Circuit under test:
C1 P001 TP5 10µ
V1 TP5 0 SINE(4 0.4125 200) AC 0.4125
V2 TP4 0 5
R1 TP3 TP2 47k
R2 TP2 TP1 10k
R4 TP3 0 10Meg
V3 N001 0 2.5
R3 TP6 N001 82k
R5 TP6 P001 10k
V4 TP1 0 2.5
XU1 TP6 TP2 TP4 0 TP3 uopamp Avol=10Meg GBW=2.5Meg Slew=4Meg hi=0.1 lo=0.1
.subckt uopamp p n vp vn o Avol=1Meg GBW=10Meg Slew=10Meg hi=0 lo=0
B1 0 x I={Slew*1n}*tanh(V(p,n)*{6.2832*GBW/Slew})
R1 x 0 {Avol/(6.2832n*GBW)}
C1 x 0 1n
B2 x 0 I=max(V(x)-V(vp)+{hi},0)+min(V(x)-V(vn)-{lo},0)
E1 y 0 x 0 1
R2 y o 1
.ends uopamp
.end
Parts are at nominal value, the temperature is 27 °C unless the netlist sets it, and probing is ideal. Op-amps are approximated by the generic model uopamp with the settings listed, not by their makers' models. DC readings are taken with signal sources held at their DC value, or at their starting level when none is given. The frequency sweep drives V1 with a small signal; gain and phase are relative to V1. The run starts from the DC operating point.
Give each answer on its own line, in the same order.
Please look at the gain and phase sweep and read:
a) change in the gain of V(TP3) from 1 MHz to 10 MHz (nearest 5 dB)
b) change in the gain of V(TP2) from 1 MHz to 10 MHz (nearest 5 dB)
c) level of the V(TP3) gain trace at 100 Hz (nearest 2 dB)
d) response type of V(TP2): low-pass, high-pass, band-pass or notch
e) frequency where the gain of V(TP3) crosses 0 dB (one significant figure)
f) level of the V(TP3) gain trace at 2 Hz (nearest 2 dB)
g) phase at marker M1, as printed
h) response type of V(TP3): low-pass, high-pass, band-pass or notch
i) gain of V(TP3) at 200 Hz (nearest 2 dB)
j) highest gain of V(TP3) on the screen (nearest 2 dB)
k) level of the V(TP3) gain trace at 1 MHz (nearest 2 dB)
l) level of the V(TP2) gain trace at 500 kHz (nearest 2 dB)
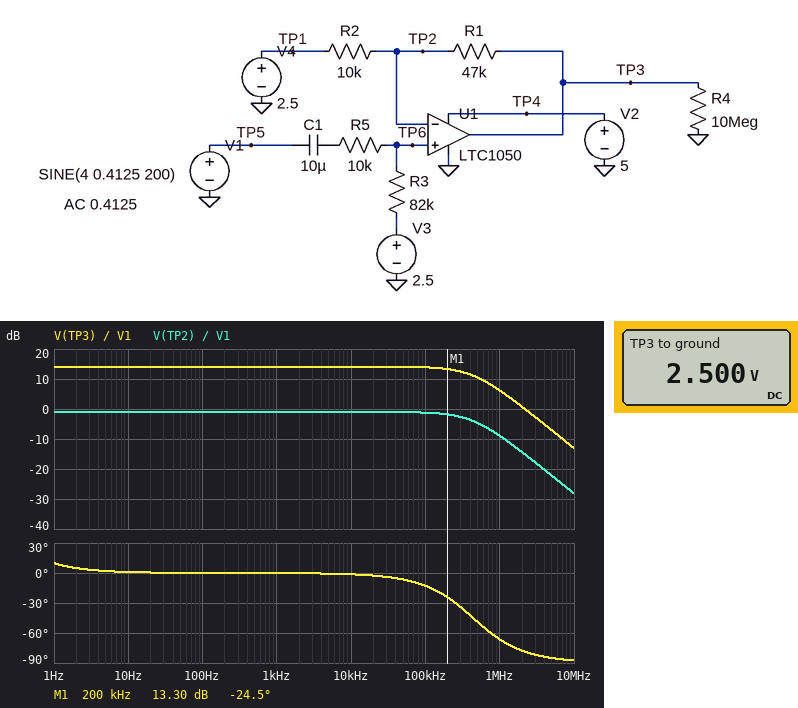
-20 dB
-20 dB
14 dB
low-pass
2 MHz
14 dB
-24.5 deg
low-pass
14 dB
14 dB
6 dB
-4 dB
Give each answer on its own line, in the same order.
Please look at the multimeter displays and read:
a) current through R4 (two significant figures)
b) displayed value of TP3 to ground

250 nA
2.500 V
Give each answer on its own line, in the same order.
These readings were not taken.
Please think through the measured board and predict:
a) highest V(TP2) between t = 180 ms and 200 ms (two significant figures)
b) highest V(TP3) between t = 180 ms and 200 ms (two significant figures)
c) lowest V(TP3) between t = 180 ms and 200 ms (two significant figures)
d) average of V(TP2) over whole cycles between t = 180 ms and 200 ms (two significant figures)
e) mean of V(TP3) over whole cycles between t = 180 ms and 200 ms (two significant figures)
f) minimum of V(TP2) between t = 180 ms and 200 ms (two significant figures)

2.9 V
4.6 V
400 mV
2.5 V
2.5 V
2.1 V
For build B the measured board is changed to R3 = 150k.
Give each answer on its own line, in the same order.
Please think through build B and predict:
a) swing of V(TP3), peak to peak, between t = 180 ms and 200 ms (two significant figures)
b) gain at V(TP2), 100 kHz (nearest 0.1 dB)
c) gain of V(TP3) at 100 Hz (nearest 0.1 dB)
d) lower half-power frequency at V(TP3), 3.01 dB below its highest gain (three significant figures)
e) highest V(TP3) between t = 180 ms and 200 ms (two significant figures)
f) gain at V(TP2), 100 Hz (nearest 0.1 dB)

4.4 V
-0.8 dB
14.6 dB
99.5 mHz
4.7 V
-0.6 dB
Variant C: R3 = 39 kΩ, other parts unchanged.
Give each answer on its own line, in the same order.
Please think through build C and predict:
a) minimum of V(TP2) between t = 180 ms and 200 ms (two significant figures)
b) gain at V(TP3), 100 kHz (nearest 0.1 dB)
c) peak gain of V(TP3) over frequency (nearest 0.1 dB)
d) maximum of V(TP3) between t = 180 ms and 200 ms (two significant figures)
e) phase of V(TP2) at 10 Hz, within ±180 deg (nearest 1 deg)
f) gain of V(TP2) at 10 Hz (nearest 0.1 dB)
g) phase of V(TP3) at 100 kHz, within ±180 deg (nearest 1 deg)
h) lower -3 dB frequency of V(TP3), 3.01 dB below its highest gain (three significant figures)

2.2 V
12.9 dB
13.1 dB
4.4 V
2 deg
-2.0 dB
-13 deg
325 mHz
